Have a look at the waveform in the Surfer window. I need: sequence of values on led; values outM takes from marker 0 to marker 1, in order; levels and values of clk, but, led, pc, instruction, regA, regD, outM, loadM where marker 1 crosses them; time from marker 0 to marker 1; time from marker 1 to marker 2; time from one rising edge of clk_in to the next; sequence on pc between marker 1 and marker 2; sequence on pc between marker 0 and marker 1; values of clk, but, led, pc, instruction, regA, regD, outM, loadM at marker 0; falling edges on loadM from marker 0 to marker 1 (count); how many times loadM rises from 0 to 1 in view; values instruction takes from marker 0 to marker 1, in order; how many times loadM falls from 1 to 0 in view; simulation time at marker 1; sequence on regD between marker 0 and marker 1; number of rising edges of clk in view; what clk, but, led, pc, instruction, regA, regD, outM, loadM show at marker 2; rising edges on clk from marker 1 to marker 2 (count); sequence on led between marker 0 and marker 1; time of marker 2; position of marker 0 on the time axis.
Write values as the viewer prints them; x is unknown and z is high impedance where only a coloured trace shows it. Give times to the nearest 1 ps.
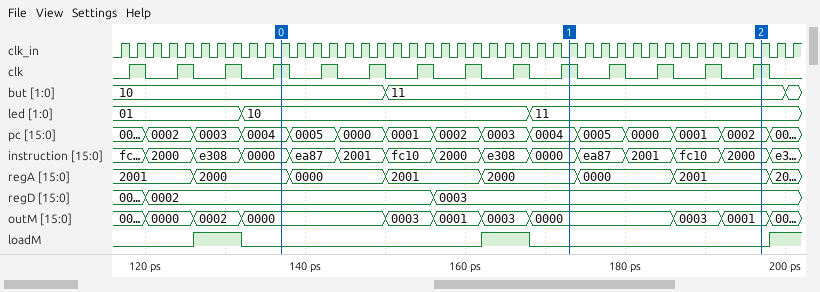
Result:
01, 10, 11
0000, 0003, 0001, 0003, 0000
clk=1, but=11, led=11, pc=0004, instruction=0000, regA=2000, regD=0003, outM=0000, loadM=0
36 ps
24 ps
2 ps
0004, 0005, 0000, 0001, 0002
0004, 0005, 0000, 0001, 0002, 0003, 0004
clk=1, but=10, led=10, pc=0004, instruction=0000, regA=2000, regD=0002, outM=0000, loadM=0
1
3
0000, ea87, 2001, fc10, 2000, e308, 0000
2
173 ps
0002, 0003
14
clk=1, but=11, led=11, pc=0002, instruction=2000, regA=2001, regD=0003, outM=0001, loadM=0
4
10, 11
197 ps
137 ps
